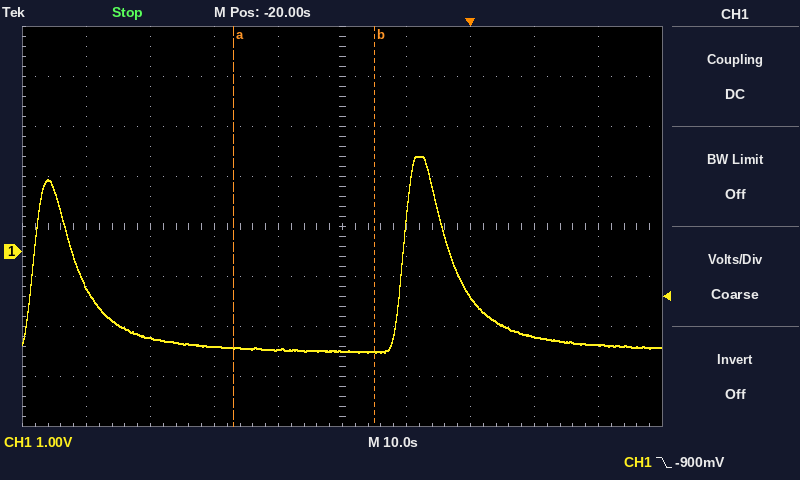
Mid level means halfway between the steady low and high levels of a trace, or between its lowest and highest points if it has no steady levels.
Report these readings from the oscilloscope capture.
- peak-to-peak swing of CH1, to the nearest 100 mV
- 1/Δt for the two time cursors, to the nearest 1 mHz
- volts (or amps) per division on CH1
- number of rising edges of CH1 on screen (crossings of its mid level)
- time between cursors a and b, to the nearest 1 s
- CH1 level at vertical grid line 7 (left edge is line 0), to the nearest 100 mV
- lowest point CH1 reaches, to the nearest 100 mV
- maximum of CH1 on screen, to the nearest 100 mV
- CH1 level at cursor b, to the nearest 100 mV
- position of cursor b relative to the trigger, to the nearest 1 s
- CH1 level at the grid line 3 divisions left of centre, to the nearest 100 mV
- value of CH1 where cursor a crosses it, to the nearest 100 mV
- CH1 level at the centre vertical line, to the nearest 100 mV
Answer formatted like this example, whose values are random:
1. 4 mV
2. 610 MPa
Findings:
1. 3.9 V
2. 45 mHz
3. 1 V
4. 2
5. 22 s
6. -900 mV
7. -2.0 V
8. 1.9 V
9. -2.0 V
10. -15 s
11. -1.7 V
12. -1.9 V
13. -2.0 V
